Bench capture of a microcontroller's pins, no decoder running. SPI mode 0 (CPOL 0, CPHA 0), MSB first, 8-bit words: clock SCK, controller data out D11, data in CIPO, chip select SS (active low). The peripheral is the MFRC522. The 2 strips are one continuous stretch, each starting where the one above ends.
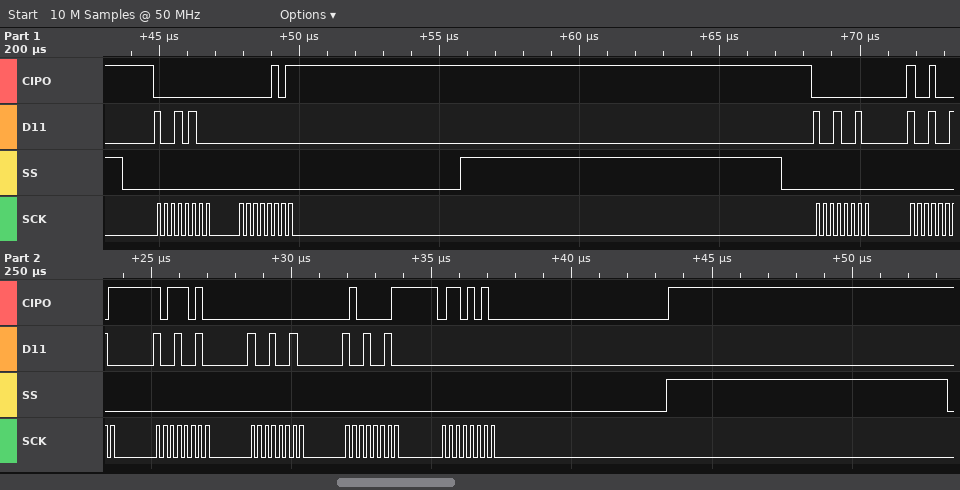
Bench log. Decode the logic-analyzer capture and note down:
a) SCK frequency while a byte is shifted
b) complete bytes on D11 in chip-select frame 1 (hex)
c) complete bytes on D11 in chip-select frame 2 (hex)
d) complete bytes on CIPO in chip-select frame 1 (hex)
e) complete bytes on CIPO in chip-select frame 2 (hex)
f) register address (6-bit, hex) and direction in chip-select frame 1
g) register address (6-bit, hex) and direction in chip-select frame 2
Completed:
4 MHz
94 00
92 92 92 92 92 00
00 05
00 91 BA 00 41 6A
0x0A read
0x09 read
